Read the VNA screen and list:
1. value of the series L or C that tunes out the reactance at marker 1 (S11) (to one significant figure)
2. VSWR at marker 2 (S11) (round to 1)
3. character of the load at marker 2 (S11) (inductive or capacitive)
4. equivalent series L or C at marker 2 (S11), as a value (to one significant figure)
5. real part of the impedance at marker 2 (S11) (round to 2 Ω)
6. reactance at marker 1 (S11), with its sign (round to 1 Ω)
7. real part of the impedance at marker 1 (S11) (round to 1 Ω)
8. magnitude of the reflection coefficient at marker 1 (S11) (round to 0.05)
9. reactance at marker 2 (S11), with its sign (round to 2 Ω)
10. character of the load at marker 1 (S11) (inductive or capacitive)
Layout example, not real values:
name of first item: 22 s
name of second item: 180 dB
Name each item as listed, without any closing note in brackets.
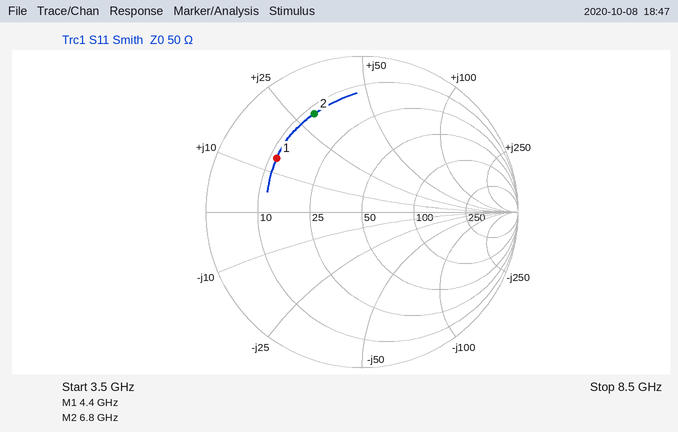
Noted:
value of the series L or C that tunes out the reactance at marker 1 (S11): 3 pF
VSWR at marker 2 (S11): 6
character of the load at marker 2 (S11): inductive
equivalent series L or C at marker 2 (S11), as a value: 700 pH
real part of the impedance at marker 2 (S11): 12 Ω
reactance at marker 1 (S11), with its sign: +14 Ω
real part of the impedance at marker 1 (S11): 12 Ω
magnitude of the reflection coefficient at marker 1 (S11): 0.65
reactance at marker 2 (S11), with its sign: +30 Ω
character of the load at marker 1 (S11): inductive
